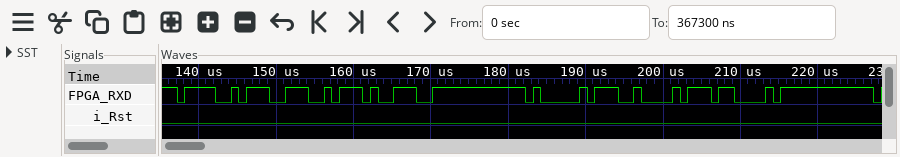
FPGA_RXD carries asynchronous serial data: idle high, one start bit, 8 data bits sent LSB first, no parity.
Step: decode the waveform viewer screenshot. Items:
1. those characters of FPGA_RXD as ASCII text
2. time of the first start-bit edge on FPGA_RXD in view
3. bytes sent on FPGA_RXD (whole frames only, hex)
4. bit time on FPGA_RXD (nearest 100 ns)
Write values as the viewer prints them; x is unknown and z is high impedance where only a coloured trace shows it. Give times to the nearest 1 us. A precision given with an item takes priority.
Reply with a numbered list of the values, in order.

1. "ON9ABC"
2. 137 us
3. 4F, 4E, 39, 41, 42, 43
4. 1000 ns
